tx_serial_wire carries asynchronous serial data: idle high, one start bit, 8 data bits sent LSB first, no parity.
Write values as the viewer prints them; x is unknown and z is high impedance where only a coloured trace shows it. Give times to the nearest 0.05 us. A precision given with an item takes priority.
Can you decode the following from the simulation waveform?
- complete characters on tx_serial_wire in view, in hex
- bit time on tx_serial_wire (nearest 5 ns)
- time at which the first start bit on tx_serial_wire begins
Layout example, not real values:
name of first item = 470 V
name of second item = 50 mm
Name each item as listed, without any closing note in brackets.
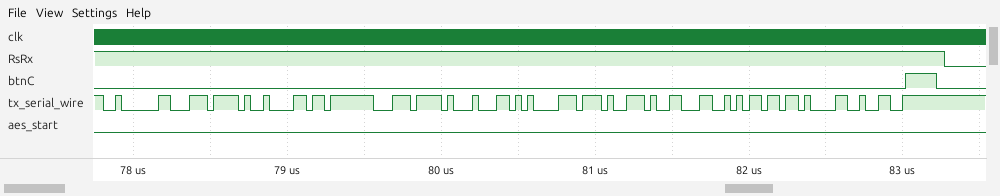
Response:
complete characters on tx_serial_wire in view, in hex = 02, DC, 09, FB, DC, 11, 85, 97, 19, 6A, 0B, 32
bit time on tx_serial_wire = 40 ns
time at which the first start bit on tx_serial_wire begins = 77.8 us
